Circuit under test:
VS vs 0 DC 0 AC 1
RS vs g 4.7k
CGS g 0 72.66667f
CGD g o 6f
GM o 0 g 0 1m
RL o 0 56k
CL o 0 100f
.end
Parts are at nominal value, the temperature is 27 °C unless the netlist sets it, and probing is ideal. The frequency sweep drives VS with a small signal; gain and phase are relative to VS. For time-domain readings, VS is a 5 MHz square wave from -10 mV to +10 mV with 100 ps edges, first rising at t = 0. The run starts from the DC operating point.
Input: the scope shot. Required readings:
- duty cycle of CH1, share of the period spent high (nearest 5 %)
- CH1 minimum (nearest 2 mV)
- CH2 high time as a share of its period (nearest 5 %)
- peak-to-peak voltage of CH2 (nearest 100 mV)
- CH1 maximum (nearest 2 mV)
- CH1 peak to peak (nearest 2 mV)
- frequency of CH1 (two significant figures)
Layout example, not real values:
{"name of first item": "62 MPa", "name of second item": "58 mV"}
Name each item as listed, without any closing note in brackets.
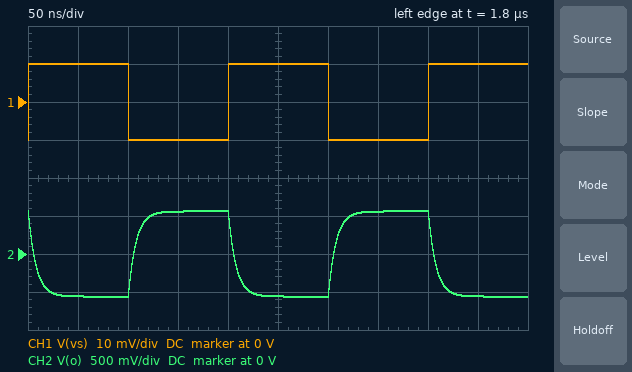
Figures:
{"duty cycle of CH1, share of the period spent high": "50 %", "CH1 minimum": "-10 mV", "CH2 high time as a share of its period": "50 %", "peak-to-peak voltage of CH2": "1.1 V", "CH1 maximum": "10 mV", "CH1 peak to peak": "20 mV", "frequency of CH1": "5.0 MHz"}
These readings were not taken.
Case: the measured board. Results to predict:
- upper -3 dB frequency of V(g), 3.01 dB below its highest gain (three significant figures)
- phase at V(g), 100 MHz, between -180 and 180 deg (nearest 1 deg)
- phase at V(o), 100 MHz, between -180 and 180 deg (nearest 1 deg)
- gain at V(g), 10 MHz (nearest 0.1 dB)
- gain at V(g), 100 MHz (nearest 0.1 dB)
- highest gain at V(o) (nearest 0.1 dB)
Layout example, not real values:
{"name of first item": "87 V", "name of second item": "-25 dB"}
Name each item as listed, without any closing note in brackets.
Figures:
{"upper -3 dB frequency of V(g), 3.01 dB below its highest gain": "263 MHz", "phase at V(g), 100 MHz, between -180 and 180 deg": "-13 deg", "phase at V(o), 100 MHz, between -180 and 180 deg": "91 deg", "gain at V(g), 10 MHz": "-0.3 dB", "gain at V(g), 100 MHz": "-2.2 dB", "highest gain at V(o)": "35.0 dB"}
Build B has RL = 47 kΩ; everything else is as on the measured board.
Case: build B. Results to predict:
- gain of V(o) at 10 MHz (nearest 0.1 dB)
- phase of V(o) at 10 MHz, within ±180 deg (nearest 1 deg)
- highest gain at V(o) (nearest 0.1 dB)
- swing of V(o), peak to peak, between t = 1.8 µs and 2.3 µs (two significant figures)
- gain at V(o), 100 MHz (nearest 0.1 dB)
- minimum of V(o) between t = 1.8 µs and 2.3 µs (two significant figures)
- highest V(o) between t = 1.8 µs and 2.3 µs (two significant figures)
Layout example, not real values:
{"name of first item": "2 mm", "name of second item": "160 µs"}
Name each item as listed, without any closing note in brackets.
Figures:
{"gain of V(o) at 10 MHz": "32.8 dB", "phase of V(o) at 10 MHz, within ±180 deg": "157 deg", "highest gain at V(o)": "33.4 dB", "swing of V(o), peak to peak, between t = 1.8 µs and 2.3 µs": "940 mV", "gain at V(o), 100 MHz": "21.0 dB", "minimum of V(o) between t = 1.8 µs and 2.3 µs": "-470 mV", "highest V(o) between t = 1.8 µs and 2.3 µs": "470 mV"}
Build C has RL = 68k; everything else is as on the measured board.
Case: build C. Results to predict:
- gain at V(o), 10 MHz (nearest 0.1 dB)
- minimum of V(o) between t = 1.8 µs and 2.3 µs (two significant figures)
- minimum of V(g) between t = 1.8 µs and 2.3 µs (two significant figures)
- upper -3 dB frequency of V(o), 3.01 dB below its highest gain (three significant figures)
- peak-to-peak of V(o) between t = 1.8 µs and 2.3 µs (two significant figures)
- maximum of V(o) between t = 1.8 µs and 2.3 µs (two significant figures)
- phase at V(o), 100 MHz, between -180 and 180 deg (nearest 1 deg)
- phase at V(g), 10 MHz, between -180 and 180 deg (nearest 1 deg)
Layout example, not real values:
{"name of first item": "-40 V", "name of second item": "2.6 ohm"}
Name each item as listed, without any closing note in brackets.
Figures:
{"gain at V(o), 10 MHz": "35.4 dB", "minimum of V(o) between t = 1.8 µs and 2.3 µs": "-680 mV", "minimum of V(g) between t = 1.8 µs and 2.3 µs": "-10 mV", "upper -3 dB frequency of V(o), 3.01 dB below its highest gain": "17.3 MHz", "peak-to-peak of V(o) between t = 1.8 µs and 2.3 µs": "1.4 V", "maximum of V(o) between t = 1.8 µs and 2.3 µs": "680 mV", "phase at V(o), 100 MHz, between -180 and 180 deg": "89 deg", "phase at V(g), 10 MHz, between -180 and 180 deg": "-7 deg"}
